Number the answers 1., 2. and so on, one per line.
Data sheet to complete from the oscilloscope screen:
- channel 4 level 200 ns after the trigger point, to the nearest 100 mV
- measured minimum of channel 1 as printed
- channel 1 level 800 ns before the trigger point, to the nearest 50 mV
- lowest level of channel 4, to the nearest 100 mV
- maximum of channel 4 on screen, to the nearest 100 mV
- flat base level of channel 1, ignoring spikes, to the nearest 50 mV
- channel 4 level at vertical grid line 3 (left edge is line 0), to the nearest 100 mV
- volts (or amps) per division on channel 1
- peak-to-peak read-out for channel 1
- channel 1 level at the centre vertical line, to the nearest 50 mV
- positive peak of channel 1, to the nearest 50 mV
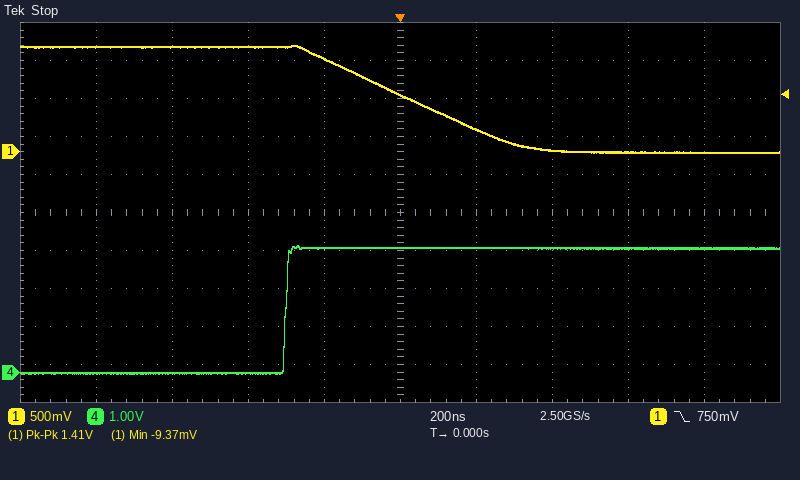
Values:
1. 3.3 V
2. -9.37 mV
3. 1.40 V
4. 0.0 V
5. 3.3 V
6. 0 mV
7. 0.0 V
8. 500 mV
9. 1.41 V
10. 750 mV
11. 1.40 V
